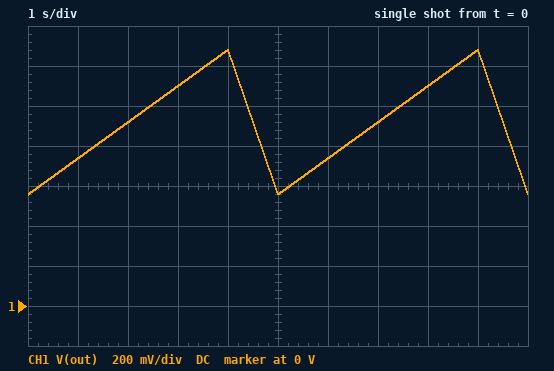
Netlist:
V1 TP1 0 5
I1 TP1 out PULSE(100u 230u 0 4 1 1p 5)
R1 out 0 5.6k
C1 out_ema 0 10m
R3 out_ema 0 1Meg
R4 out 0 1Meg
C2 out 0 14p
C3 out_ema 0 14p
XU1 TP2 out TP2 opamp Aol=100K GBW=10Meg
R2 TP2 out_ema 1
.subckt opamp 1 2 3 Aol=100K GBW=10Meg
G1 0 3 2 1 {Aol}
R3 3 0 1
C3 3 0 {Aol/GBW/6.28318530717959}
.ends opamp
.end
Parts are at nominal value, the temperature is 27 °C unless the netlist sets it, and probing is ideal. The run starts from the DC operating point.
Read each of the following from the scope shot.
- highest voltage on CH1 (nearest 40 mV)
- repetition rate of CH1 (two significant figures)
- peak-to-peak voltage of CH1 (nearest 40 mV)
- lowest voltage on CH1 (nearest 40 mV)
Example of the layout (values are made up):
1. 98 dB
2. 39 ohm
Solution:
1. 1.28 V
2. 200 mHz
3. 720 mV
4. 560 mV
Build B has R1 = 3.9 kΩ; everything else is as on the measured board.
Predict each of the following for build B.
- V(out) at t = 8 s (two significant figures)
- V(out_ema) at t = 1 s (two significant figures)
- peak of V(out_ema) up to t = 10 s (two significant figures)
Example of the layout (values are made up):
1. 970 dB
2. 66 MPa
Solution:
1. 770 mV
2. 510 mV
3. 890 mV
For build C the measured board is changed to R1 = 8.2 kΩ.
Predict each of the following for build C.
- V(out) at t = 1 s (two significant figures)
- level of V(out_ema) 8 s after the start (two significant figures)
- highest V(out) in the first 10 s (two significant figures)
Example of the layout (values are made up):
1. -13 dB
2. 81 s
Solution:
1. 1.1 V
2. 1.6 V
3. 1.9 V
